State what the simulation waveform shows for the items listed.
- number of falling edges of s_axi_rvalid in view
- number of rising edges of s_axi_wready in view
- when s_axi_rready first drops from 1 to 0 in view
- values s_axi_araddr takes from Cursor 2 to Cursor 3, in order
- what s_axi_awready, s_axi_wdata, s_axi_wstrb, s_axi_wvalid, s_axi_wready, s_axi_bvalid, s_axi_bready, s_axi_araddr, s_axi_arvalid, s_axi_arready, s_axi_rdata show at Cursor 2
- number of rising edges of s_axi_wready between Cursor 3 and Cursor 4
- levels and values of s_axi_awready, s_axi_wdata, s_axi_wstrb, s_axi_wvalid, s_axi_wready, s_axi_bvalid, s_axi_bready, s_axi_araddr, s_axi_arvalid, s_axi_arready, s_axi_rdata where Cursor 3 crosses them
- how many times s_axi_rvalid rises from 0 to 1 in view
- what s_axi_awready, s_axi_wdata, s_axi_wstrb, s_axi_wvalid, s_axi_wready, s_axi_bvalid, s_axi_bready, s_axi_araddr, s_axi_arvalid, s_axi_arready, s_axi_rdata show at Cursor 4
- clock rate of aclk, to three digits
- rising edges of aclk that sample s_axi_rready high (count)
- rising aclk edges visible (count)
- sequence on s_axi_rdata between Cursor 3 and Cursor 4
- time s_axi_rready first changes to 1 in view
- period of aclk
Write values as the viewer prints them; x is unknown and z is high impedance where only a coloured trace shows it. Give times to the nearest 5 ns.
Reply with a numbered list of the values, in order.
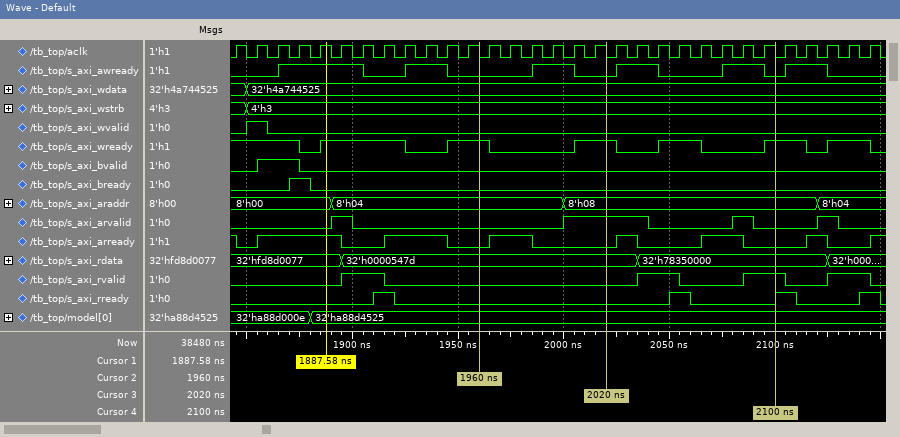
1. 4
2. 6
3. 1920 ns
4. 8'h04, 8'h08
5. s_axi_awready=0, s_axi_wdata=32'h4a744525, s_axi_wstrb=4'h3, s_axi_wvalid=0, s_axi_wready=1, s_axi_bvalid=0, s_axi_bready=0, s_axi_araddr=8'h04, s_axi_arvalid=0, s_axi_arready=0, s_axi_rdata=32'h0000547d
6. 2
7. s_axi_awready=0, s_axi_wdata=32'h4a744525, s_axi_wstrb=4'h3, s_axi_wvalid=0, s_axi_wready=1, s_axi_bvalid=0, s_axi_bready=0, s_axi_araddr=8'h08, s_axi_arvalid=1, s_axi_arready=0, s_axi_rdata=32'h0000547d
8. 4
9. s_axi_awready=0, s_axi_wdata=32'h4a744525, s_axi_wstrb=4'h3, s_axi_wvalid=0, s_axi_wready=1, s_axi_bvalid=0, s_axi_bready=0, s_axi_araddr=8'h08, s_axi_arvalid=0, s_axi_arready=0, s_axi_rdata=32'h78350000
10. 100 MHz
11. 4
12. 31
13. 32'h0000547d, 32'h78350000
14. 1910 ns
15. 10 ns
